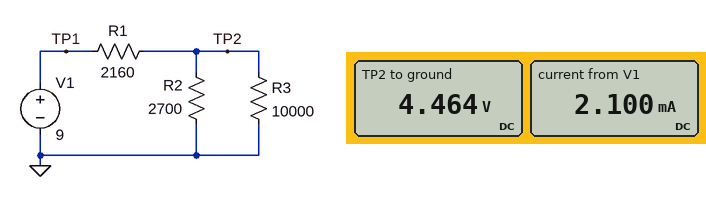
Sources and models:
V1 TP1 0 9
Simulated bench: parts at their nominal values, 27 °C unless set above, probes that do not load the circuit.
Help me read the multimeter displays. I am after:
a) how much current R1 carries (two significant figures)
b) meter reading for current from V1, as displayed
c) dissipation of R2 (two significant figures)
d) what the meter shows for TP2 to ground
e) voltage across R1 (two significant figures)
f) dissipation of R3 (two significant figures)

2.1 mA
2.100 mA
7.4 mW
4.464 V
4.5 V
2.0 mW
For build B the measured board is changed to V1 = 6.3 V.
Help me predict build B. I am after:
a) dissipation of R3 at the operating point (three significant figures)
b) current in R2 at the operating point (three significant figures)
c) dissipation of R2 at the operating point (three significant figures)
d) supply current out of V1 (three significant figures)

977 µW
1.16 mA
3.62 mW
1.47 mA
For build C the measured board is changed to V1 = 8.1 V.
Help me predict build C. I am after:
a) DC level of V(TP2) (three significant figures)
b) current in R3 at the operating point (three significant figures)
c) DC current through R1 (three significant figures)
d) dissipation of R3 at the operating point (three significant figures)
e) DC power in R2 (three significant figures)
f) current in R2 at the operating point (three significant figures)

4.02 V
402 µA
1.89 mA
1.61 mW
5.98 mW
1.49 mA
